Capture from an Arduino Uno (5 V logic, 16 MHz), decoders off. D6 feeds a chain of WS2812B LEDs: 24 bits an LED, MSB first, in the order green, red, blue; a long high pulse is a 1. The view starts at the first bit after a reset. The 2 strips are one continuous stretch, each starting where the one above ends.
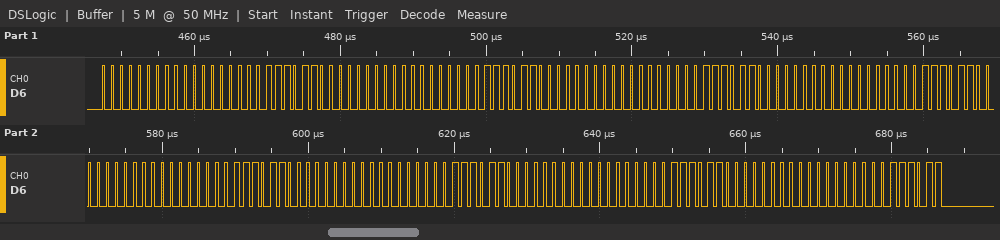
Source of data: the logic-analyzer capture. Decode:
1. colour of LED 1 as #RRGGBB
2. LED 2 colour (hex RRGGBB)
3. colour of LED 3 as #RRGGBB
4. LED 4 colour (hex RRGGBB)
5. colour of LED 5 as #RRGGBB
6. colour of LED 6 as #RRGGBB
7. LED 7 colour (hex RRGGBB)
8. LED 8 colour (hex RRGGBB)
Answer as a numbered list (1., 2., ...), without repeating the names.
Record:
1. #00003B
2. #00003B
3. #00003B
4. #00003B
5. #00003B
6. #00003B
7. #00003B
8. #00003B
